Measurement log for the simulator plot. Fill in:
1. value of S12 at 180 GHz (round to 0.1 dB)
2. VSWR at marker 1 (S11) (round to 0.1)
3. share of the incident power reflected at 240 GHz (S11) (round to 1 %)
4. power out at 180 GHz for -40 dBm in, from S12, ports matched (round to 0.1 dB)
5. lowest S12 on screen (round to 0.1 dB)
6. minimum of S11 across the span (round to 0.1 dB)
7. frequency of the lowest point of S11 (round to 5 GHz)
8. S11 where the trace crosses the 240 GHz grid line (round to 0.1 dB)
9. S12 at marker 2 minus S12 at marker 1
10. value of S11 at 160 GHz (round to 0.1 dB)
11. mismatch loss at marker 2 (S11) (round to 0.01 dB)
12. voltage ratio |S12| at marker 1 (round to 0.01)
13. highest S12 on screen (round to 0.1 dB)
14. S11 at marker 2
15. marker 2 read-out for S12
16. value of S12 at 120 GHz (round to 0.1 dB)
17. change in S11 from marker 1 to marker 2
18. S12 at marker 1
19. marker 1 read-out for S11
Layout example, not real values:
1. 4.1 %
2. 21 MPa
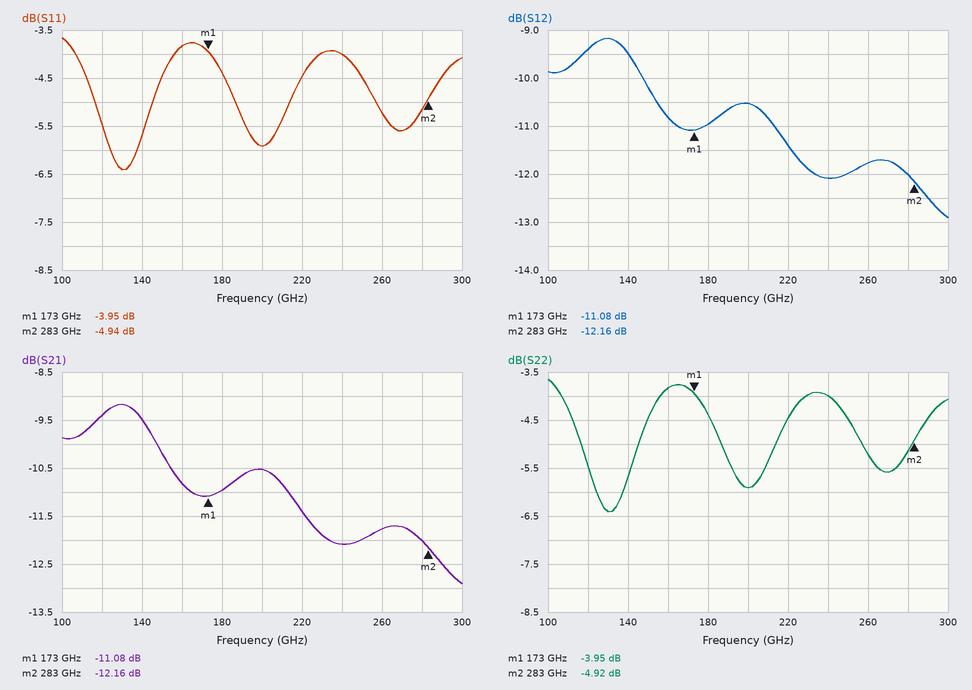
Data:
1. -11.0 dB
2. 4.5
3. 40 %
4. -51.0 dBm
5. -12.9 dB
6. -6.4 dB
7. 130 GHz
8. -4.0 dB
9. -1.08 dB
10. -3.8 dB
11. 1.68 dB
12. 0.28
13. -9.2 dB
14. -4.94 dB
15. -12.16 dB
16. -9.4 dB
17. -0.99 dB
18. -11.08 dB
19. -3.95 dB
